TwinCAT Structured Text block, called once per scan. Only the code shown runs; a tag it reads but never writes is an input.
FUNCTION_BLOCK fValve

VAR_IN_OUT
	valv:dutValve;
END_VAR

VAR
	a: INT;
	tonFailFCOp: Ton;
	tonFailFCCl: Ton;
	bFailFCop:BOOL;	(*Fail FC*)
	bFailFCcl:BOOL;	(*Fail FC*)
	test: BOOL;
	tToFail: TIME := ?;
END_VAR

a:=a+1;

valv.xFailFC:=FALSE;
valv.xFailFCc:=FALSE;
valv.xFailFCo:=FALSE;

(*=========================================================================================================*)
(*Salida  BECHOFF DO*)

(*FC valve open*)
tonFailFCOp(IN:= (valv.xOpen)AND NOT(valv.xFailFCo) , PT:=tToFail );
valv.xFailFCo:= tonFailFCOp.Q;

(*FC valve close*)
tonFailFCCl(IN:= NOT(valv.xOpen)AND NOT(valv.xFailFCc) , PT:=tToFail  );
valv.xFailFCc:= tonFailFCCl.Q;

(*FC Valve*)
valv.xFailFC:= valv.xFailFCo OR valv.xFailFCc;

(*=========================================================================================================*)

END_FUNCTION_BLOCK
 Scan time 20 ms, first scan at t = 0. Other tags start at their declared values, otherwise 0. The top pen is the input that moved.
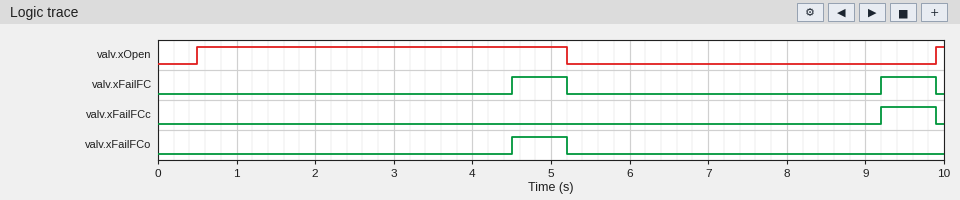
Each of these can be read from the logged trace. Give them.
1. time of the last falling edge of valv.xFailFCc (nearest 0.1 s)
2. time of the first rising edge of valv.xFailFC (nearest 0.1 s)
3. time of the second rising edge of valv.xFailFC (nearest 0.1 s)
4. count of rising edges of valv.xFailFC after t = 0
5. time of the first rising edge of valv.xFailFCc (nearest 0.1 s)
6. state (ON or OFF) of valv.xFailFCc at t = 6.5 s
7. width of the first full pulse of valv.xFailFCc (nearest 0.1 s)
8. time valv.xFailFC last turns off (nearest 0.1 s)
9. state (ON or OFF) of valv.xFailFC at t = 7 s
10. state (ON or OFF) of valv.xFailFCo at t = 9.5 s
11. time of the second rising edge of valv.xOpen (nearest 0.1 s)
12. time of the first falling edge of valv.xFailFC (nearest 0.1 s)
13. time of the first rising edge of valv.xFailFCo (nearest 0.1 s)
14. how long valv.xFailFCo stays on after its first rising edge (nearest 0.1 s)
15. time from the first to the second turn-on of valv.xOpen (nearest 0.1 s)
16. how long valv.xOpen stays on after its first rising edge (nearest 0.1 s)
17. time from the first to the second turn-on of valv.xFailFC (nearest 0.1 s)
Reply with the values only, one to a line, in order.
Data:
9.9 s
4.5 s
9.2 s
2
9.2 s
OFF
0.7 s
9.9 s
OFF
OFF
9.9 s
5.2 s
4.5 s
0.7 s
9.4 s
4.7 s
4.7 s
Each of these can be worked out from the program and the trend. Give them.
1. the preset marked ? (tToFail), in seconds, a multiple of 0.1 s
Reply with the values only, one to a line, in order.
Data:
4.0 s
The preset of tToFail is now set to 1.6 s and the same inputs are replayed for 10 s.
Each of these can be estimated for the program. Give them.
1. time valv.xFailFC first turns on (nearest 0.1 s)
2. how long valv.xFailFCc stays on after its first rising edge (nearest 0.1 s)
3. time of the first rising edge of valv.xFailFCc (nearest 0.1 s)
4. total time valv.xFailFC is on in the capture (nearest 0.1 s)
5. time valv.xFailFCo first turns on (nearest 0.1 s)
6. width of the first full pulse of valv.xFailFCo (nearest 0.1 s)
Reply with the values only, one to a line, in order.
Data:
2.1 s
3.1 s
6.8 s
6.2 s
2.1 s
3.1 s
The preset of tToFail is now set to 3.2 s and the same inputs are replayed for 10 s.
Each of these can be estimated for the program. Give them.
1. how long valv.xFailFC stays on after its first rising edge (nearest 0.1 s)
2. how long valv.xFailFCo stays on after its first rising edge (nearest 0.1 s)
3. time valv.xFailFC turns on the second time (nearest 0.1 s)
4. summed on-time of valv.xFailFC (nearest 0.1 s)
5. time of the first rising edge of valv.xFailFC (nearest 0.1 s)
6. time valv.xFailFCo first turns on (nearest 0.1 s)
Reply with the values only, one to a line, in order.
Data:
1.5 s
1.5 s
8.4 s
3.0 s
3.7 s
3.7 s
